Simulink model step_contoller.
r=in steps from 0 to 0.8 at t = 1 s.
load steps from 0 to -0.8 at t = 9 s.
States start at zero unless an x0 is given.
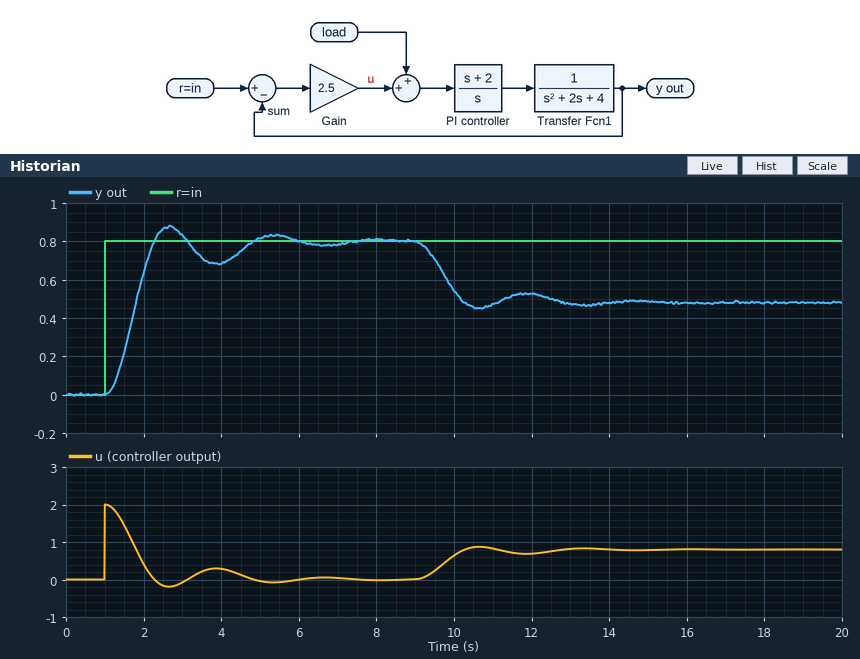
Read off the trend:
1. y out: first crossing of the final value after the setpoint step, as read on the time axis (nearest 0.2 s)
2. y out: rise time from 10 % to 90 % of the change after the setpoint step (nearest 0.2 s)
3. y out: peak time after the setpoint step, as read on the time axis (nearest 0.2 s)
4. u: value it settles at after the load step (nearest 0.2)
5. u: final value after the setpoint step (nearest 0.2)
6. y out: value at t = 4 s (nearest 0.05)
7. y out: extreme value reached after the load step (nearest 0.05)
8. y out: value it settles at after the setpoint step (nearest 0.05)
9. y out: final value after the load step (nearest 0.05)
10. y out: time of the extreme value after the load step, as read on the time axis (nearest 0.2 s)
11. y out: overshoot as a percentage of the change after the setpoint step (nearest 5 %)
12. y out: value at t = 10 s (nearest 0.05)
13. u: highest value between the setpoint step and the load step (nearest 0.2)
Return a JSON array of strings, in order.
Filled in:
["2.2 s", "0.8 s", "2.6 s", "0.8", "0.0", "0.70", "0.45", "0.80", "0.50", "10.6 s", "10 %", "0.55", "2.0"]
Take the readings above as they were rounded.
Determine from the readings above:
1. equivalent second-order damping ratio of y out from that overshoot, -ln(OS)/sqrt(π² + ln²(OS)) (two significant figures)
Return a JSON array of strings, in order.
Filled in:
["0.59"]
